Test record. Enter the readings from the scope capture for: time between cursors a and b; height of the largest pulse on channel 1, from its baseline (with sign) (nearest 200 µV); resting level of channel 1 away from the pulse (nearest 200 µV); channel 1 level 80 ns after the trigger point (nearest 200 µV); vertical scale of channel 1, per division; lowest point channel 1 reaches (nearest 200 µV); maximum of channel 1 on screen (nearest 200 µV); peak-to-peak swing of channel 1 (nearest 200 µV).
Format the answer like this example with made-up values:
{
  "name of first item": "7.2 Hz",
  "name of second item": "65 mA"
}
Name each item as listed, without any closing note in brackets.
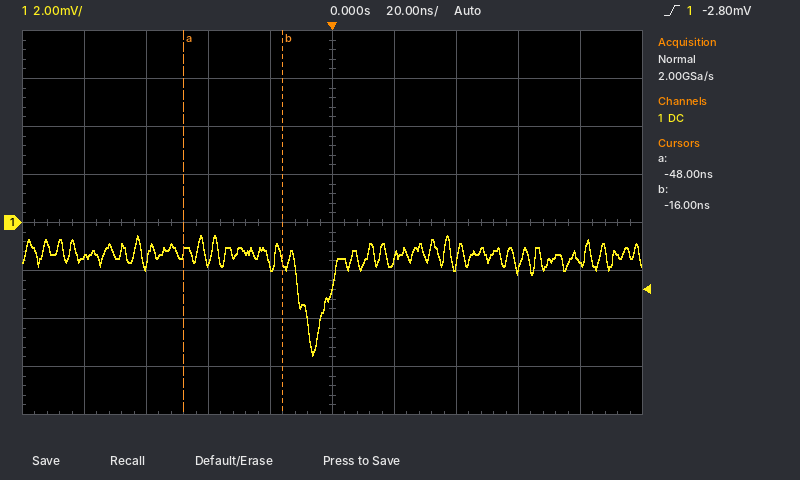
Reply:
{
  "time between cursors a and b": "32 ns",
  "height of the largest pulse on channel 1, from its baseline (with sign)": "-4.2 mV",
  "resting level of channel 1 away from the pulse": "-1.4 mV",
  "channel 1 level 80 ns after the trigger point": "-1.6 mV",
  "vertical scale of channel 1, per division": "2 mV",
  "lowest point channel 1 reaches": "-5.6 mV",
  "maximum of channel 1 on screen": "-600 µV",
  "peak-to-peak swing of channel 1": "5.0 mV"
}
